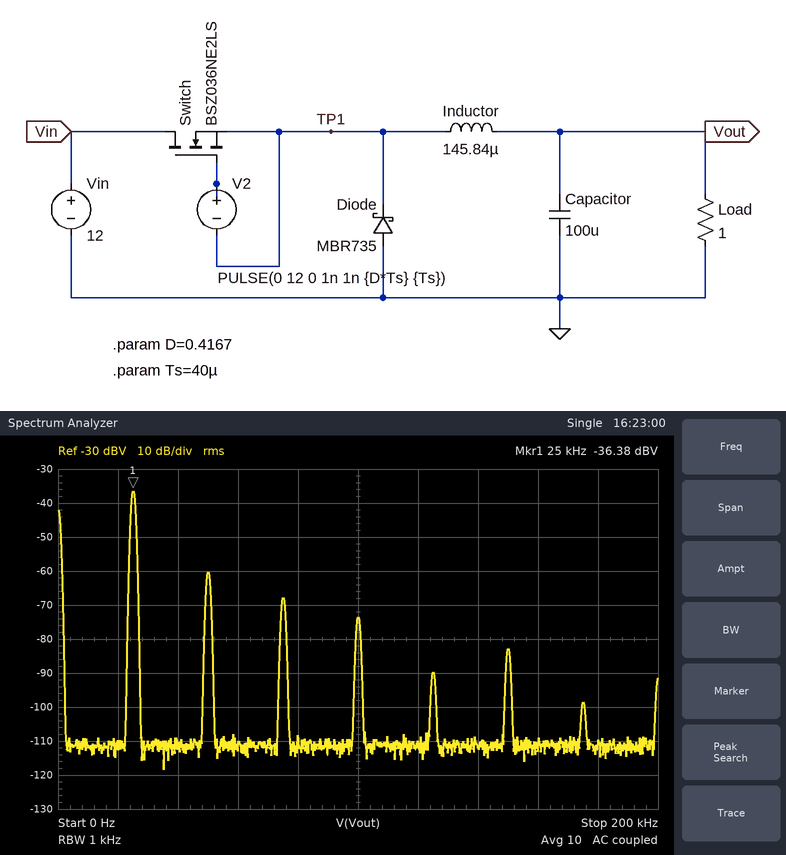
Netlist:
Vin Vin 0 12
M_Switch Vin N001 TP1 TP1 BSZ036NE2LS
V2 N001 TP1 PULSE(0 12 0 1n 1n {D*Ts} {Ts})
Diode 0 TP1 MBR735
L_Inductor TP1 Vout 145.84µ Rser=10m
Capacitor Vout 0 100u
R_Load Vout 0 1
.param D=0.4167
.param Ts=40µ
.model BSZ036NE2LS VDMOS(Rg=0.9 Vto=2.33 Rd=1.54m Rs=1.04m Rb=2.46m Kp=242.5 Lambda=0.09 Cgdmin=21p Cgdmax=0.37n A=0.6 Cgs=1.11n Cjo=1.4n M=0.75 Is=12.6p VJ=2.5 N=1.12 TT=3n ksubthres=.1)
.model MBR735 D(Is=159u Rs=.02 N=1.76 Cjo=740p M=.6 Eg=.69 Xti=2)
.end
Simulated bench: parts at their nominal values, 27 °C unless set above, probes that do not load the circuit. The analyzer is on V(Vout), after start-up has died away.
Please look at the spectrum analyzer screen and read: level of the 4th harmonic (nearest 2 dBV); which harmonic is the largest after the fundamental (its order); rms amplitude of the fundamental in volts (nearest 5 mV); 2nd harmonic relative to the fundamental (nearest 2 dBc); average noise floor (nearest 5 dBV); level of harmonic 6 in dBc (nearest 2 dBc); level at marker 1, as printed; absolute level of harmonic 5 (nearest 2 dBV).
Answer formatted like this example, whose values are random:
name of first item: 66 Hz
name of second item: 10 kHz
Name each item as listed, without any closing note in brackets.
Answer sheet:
level of the 4th harmonic: -74 dBV
which harmonic is the largest after the fundamental: 2
rms amplitude of the fundamental in volts: 15 mV
2nd harmonic relative to the fundamental: -24 dBc
average noise floor: -110 dBV
level of harmonic 6 in dBc: -46 dBc
level at marker 1, as printed: -36.38 dBV
absolute level of harmonic 5: -90 dBV
